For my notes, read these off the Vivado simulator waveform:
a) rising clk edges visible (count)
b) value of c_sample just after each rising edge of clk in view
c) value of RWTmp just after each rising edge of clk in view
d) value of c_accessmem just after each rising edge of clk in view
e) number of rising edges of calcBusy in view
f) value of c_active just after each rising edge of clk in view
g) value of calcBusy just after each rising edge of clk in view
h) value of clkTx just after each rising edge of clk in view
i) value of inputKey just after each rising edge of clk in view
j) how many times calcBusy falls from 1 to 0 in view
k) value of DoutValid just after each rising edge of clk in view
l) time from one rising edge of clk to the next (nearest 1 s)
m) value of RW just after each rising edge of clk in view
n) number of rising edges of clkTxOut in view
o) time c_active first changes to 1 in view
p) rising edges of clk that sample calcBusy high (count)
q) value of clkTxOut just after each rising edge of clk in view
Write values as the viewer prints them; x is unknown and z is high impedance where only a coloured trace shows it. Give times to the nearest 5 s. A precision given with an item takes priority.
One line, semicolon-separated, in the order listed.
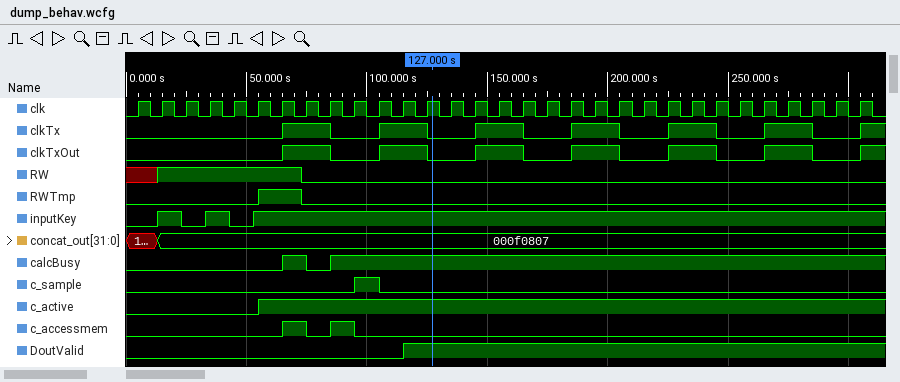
31; 0 0 0 0 0 0 0 0 0 1 0 0 0 0 0 0 0 0 0 0 0 0 0 0 0 0 0 0 0 0 0; 0 0 0 0 0 1 1 0 0 0 0 0 0 0 0 0 0 0 0 0 0 0 0 0 0 0 0 0 0 0 0; 0 0 0 0 0 0 1 0 1 0 0 0 0 0 0 0 0 0 0 0 0 0 0 0 0 0 0 0 0 0 0; 2; 0 0 0 0 0 1 1 1 1 1 1 1 1 1 1 1 1 1 1 1 1 1 1 1 1 1 1 1 1 1 1; 0 0 0 0 0 0 1 0 1 1 1 1 1 1 1 1 1 1 1 1 1 1 1 1 1 1 1 1 1 1 1; 0 0 0 0 0 0 1 1 0 0 1 1 0 0 1 1 0 0 1 1 0 0 1 1 0 0 1 1 0 0 1; 0 1 0 1 0 1 1 1 1 1 1 1 1 1 1 1 1 1 1 1 1 1 1 1 1 1 1 1 1 1 1; 1; 0 0 0 0 0 0 0 0 0 0 0 1 1 1 1 1 1 1 1 1 1 1 1 1 1 1 1 1 1 1 1; 10 s; x 1 1 1 1 1 1 0 0 0 0 0 0 0 0 0 0 0 0 0 0 0 0 0 0 0 0 0 0 0 0; 7; 55 s; 23; 0 0 0 0 0 0 1 1 0 0 1 1 0 0 1 1 0 0 1 1 0 0 1 1 0 0 1 1 0 0 1
